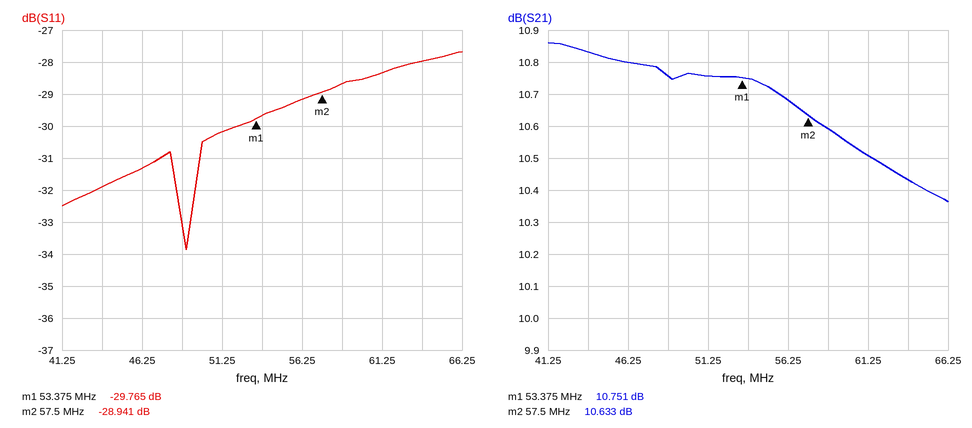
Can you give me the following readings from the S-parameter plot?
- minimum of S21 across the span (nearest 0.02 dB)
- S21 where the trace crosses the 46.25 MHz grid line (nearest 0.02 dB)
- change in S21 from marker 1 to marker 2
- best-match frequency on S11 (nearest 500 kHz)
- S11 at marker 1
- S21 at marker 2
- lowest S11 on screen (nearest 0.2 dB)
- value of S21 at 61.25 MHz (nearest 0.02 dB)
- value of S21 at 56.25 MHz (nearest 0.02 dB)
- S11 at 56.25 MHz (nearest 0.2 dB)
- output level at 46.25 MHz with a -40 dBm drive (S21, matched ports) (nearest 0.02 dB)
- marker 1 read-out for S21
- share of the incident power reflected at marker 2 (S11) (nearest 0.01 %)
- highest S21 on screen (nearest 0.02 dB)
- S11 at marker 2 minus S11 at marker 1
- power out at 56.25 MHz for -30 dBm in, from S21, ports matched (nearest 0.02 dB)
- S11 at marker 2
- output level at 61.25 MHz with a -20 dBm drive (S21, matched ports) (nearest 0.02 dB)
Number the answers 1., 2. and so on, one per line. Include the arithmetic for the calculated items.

1. 10.36 dB
2. 10.80 dB
3. 10.633 − (10.751) = -0.118 dB
4. 49.0 MHz
5. -29.765 dB
6. 10.633 dB
7. -33.8 dB
8. 10.50 dB
9. 10.68 dB
10. -29.2 dB
11. -40 dBm + (10.80 dB) = -29.20 dBm
12. 10.751 dB
13. 10^(-28.941/10) ≈ 0.13 %
14. 10.86 dB
15. -28.941 − (-29.765) = 0.824 dB
16. -30 dBm + (10.68 dB) = -19.32 dBm
17. -28.941 dB
18. -20 dBm + (10.50 dB) = -9.50 dBm
